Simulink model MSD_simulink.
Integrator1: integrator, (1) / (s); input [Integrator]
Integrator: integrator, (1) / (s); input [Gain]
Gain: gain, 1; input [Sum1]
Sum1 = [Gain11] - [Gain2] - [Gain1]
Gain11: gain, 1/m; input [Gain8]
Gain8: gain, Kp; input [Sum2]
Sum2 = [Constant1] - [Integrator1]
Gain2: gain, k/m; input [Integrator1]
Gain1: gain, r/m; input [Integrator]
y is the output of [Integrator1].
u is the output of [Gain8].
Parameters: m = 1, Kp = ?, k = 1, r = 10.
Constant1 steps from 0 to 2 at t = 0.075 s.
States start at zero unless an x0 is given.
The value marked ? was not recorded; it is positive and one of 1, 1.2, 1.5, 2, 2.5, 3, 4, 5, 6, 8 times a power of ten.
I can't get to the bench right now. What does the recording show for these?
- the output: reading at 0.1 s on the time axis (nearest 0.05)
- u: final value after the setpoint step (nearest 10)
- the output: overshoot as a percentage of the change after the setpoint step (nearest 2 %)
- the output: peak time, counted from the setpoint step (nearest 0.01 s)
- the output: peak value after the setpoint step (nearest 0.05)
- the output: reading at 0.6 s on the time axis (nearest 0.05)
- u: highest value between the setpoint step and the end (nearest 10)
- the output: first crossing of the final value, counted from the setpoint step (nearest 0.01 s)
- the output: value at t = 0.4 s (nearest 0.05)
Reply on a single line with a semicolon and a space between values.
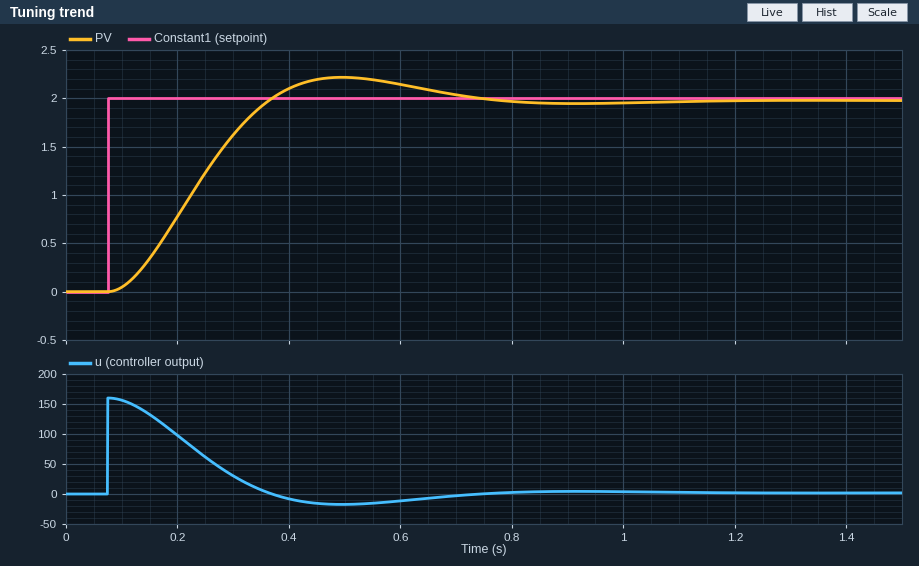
0.05; 0; 12 %; 0.42 s; 2.20; 2.15; 160; 0.29 s; 2.10
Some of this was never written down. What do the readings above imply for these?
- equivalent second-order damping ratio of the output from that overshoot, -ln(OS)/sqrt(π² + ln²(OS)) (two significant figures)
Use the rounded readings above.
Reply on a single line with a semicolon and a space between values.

0.56
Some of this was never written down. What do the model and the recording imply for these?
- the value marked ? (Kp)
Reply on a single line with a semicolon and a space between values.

80
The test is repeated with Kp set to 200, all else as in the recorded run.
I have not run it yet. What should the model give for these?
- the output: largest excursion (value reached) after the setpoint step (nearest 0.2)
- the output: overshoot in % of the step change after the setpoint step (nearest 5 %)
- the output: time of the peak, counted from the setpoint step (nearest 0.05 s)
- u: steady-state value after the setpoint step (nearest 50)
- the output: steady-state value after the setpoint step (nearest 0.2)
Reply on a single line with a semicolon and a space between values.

2.6; 30 %; 0.25 s; 0; 2.0
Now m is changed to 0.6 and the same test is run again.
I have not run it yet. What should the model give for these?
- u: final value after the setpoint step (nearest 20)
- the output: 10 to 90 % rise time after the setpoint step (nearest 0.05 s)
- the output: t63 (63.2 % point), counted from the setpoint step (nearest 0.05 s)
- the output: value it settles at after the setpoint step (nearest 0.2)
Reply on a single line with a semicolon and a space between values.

0; 0.20 s; 0.15 s; 2.0
